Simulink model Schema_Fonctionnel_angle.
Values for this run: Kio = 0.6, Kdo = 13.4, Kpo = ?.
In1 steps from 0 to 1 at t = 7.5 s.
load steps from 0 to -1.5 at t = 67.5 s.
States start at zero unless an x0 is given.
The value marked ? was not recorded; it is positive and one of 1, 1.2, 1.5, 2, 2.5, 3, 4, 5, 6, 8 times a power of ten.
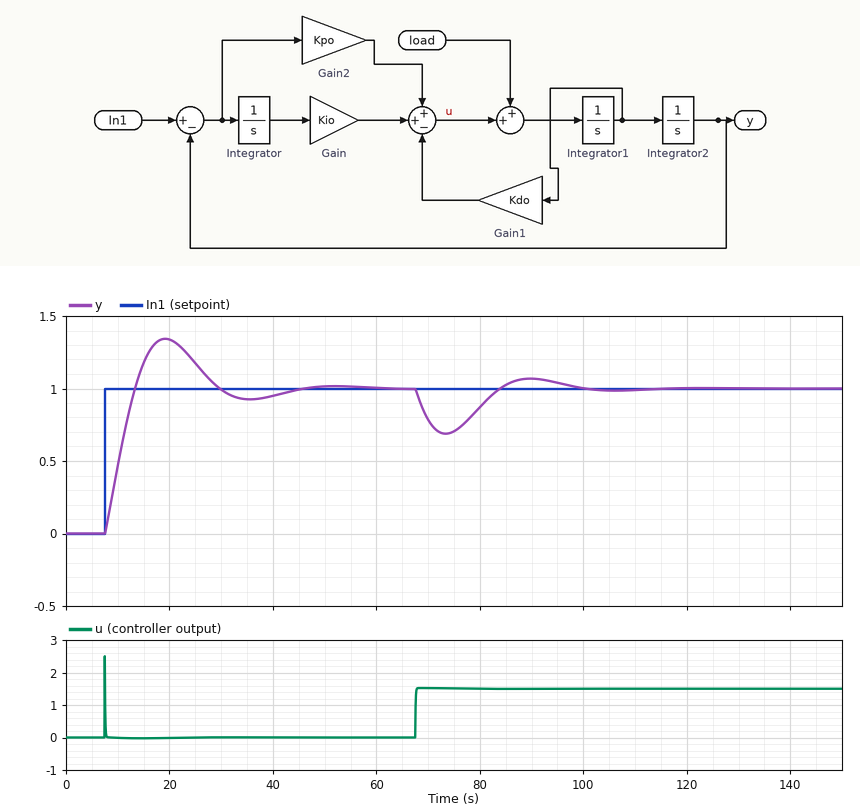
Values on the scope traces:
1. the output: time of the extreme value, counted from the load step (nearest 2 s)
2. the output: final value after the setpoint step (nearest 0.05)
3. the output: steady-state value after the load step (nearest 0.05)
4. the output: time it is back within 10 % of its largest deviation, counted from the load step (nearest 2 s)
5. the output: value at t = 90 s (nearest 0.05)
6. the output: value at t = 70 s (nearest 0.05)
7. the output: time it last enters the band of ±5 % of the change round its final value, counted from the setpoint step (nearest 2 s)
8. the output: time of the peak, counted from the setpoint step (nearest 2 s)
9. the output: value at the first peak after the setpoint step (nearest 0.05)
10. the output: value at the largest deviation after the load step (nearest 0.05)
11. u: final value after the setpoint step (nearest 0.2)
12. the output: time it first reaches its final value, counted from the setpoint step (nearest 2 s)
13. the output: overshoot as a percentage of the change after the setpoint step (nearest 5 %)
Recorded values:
6 s
1.00
1.00
28 s
1.05
0.80
32 s
12 s
1.35
0.70
0.0
6 s
35 %
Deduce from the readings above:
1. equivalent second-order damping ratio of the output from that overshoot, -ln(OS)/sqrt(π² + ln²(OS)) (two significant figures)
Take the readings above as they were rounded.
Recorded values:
0.32
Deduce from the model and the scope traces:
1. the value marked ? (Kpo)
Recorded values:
2.5
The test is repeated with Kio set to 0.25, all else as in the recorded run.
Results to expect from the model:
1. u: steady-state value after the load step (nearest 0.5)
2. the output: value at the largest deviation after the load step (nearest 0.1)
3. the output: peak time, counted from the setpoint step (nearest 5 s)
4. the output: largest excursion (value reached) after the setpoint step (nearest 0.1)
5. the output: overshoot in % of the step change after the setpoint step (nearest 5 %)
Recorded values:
1.5
0.6
15 s
1.2
20 %
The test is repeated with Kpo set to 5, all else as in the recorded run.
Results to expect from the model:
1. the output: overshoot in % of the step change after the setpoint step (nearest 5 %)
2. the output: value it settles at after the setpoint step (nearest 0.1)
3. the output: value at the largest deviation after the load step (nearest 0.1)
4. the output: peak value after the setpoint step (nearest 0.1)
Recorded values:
15 %
1.0
0.8
1.2
